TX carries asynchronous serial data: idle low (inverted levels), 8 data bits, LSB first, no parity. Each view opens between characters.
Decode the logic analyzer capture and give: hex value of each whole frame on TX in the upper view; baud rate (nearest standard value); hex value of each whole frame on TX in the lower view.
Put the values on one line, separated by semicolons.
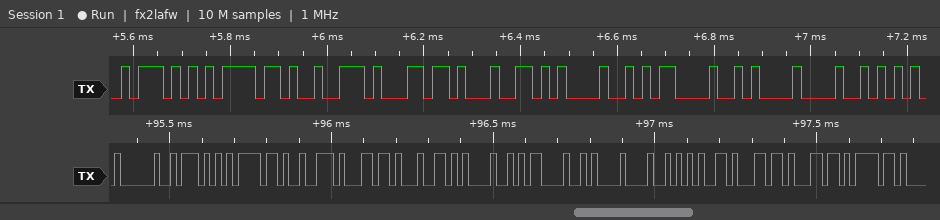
51, 21, 1B, 27, 37, BD, E5, EB, 6F; 57600 baud; BF, 51, 21, 1B, 27, 37, BD, E5, EB, 6F, 35, 27, 27, 21
